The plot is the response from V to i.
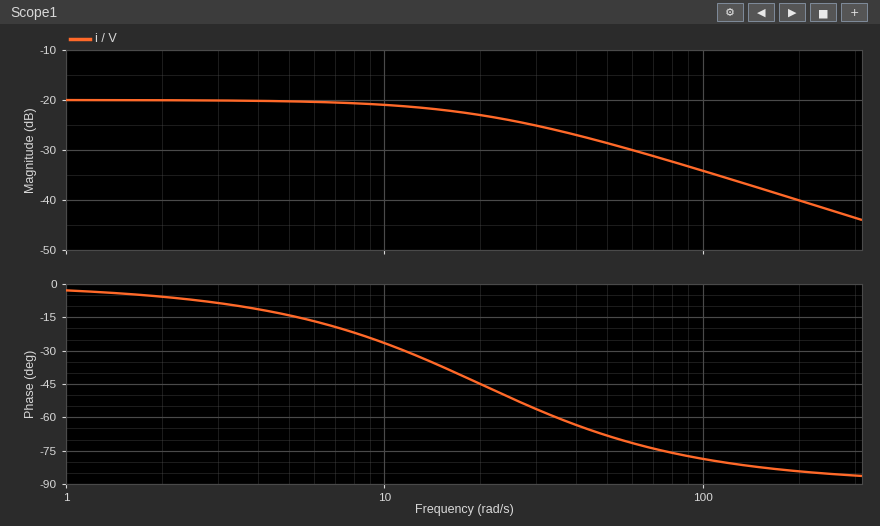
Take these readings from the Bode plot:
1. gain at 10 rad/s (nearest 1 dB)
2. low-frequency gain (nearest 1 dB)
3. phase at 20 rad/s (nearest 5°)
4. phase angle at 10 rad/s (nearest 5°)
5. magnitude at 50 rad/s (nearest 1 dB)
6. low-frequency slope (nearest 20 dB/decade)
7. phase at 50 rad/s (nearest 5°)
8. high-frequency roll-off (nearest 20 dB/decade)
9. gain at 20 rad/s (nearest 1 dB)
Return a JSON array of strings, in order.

["-21 dB", "-20 dB", "-45°", "-25°", "-29 dB", "0 dB/decade", "-70°", "-20 dB/decade", "-23 dB"]
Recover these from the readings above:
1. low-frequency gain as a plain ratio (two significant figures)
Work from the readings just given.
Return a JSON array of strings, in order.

["0.10"]
